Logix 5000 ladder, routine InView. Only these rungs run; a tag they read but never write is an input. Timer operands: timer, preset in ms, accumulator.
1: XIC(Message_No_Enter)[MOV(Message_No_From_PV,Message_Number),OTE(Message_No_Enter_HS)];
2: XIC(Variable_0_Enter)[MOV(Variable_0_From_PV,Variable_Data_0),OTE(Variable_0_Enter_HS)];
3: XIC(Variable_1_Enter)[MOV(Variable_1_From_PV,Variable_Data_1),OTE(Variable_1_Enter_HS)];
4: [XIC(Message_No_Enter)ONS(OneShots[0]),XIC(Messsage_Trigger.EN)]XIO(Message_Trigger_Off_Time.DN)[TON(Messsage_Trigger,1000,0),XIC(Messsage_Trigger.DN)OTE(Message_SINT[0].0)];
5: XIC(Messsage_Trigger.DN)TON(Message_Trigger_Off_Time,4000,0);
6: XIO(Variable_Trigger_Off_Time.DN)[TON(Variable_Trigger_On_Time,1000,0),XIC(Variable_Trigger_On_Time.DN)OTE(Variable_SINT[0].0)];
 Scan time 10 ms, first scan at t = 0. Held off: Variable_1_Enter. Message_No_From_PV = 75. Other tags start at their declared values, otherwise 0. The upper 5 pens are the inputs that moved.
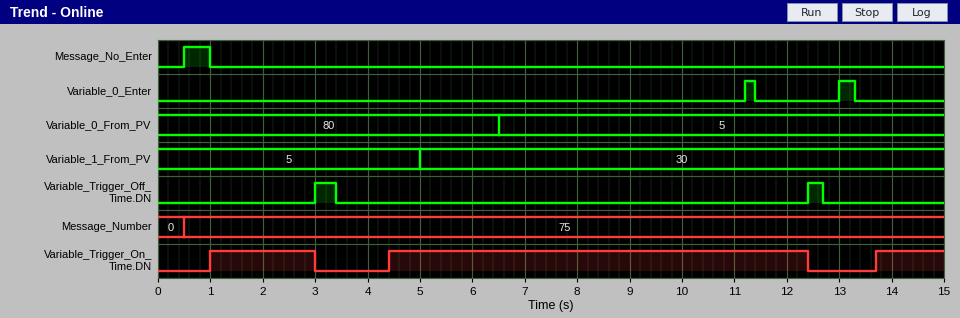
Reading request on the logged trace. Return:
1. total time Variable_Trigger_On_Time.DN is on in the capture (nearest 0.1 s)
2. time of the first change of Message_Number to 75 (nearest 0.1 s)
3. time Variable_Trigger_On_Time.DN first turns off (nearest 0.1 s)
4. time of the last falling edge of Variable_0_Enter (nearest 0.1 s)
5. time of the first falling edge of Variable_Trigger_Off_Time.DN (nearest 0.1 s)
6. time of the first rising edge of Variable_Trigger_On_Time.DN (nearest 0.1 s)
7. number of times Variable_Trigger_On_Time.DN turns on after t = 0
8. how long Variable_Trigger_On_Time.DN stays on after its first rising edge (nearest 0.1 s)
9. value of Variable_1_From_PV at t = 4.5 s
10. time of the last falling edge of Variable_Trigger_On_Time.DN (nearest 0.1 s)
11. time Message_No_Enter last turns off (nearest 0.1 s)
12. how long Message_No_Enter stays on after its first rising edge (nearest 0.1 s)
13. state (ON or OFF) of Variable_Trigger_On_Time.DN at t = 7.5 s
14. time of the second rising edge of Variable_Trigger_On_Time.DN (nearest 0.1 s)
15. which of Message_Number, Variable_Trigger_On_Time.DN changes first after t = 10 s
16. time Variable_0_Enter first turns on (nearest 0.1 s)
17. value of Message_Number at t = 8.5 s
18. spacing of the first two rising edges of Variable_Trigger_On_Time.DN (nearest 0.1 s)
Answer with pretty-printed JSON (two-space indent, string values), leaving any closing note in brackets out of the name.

{
  "total time Variable_Trigger_On_Time.DN is on in the capture": "11.3 s",
  "time of the first change of Message_Number to 75": "0.5 s",
  "time Variable_Trigger_On_Time.DN first turns off": "3.0 s",
  "time of the last falling edge of Variable_0_Enter": "13.3 s",
  "time of the first falling edge of Variable_Trigger_Off_Time.DN": "3.4 s",
  "time of the first rising edge of Variable_Trigger_On_Time.DN": "1.0 s",
  "number of times Variable_Trigger_On_Time.DN turns on after t = 0": "3",
  "how long Variable_Trigger_On_Time.DN stays on after its first rising edge": "2.0 s",
  "value of Variable_1_From_PV at t = 4.5 s": "5",
  "time of the last falling edge of Variable_Trigger_On_Time.DN": "12.4 s",
  "time Message_No_Enter last turns off": "1.0 s",
  "how long Message_No_Enter stays on after its first rising edge": "0.5 s",
  "state (ON or OFF) of Variable_Trigger_On_Time.DN at t = 7.5 s": "ON",
  "time of the second rising edge of Variable_Trigger_On_Time.DN": "4.4 s",
  "which of Message_Number, Variable_Trigger_On_Time.DN changes first after t = 10 s": "Variable_Trigger_On_Time.DN",
  "time Variable_0_Enter first turns on": "11.2 s",
  "value of Message_Number at t = 8.5 s": "75",
  "spacing of the first two rising edges of Variable_Trigger_On_Time.DN": "3.4 s"
}
